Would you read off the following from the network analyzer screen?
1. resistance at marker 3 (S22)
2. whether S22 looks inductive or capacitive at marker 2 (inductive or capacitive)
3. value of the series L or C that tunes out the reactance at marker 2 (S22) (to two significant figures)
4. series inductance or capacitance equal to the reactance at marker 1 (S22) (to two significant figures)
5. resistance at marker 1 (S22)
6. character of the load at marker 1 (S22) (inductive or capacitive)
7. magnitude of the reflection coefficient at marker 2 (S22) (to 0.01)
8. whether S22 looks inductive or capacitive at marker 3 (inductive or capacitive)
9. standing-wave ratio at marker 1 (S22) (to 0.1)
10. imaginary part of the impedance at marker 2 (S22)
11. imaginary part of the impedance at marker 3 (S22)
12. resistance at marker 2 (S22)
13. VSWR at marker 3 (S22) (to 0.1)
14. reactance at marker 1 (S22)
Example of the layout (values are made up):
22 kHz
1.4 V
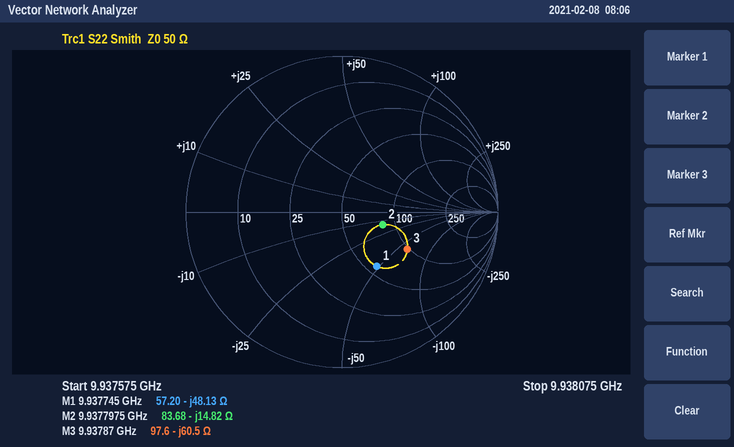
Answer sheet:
97.6 Ω
capacitive
240 pH
330 fF
57.20 Ω
capacitive
0.27
capacitive
2.4
-14.82 Ω
-60.5 Ω
83.68 Ω
2.9
-48.13 Ω
